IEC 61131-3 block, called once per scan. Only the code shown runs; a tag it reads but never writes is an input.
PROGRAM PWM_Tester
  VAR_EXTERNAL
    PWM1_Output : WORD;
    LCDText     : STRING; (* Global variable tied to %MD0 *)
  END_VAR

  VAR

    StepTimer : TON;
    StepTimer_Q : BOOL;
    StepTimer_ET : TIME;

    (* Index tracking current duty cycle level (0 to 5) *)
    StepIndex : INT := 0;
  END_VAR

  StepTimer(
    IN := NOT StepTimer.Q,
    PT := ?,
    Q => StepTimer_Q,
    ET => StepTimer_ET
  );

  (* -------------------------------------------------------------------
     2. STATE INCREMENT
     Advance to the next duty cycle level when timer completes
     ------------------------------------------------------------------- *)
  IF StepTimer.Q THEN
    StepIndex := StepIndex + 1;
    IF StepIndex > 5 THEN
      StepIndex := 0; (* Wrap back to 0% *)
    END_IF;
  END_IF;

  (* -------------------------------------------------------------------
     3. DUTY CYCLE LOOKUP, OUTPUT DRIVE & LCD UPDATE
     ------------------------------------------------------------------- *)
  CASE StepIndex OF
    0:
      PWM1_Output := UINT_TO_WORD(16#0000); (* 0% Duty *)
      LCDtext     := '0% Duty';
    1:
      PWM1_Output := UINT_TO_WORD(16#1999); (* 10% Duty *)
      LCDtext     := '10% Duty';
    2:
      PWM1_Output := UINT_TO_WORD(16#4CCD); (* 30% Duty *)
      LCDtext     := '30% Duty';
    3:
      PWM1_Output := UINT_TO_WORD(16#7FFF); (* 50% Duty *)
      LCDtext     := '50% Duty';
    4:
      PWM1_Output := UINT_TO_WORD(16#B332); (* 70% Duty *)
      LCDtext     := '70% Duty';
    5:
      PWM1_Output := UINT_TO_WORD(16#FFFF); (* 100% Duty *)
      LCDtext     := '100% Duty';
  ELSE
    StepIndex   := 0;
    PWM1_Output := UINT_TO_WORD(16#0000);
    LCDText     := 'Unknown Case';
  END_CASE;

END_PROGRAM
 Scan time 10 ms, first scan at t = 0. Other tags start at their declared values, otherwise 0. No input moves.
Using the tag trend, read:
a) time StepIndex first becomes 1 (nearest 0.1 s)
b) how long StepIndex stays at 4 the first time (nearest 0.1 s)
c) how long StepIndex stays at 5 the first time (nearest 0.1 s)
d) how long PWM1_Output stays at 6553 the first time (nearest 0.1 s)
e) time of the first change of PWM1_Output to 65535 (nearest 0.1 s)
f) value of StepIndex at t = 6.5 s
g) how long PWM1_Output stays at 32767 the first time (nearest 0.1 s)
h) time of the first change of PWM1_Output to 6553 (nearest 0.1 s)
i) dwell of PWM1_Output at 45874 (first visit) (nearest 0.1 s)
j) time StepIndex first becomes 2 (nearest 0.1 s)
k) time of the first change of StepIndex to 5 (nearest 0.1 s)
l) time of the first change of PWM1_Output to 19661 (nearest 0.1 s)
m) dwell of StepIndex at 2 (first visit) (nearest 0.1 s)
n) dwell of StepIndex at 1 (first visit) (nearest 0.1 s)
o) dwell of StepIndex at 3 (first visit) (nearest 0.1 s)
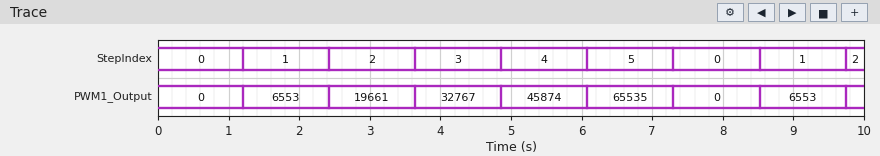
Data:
1.2 s
1.2 s
1.2 s
1.2 s
6.1 s
5
1.2 s
1.2 s
1.2 s
2.4 s
6.1 s
2.4 s
1.2 s
1.2 s
1.2 s
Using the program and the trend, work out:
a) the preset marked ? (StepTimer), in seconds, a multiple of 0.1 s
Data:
1.2 s
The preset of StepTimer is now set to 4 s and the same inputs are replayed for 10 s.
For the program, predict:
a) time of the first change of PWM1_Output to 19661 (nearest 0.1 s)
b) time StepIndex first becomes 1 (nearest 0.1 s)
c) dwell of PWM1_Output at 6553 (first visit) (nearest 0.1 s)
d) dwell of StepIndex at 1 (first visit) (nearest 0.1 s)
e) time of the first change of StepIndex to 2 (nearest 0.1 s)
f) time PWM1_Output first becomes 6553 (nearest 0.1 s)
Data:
8.0 s
4.0 s
4.0 s
4.0 s
8.0 s
4.0 s
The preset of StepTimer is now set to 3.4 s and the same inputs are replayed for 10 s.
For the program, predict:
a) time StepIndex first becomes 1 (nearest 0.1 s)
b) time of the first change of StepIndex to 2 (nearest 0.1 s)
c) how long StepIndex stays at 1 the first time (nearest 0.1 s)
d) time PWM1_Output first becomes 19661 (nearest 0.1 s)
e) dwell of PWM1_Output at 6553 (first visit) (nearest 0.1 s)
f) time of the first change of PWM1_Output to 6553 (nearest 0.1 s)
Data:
3.4 s
6.8 s
3.4 s
6.8 s
3.4 s
3.4 s
